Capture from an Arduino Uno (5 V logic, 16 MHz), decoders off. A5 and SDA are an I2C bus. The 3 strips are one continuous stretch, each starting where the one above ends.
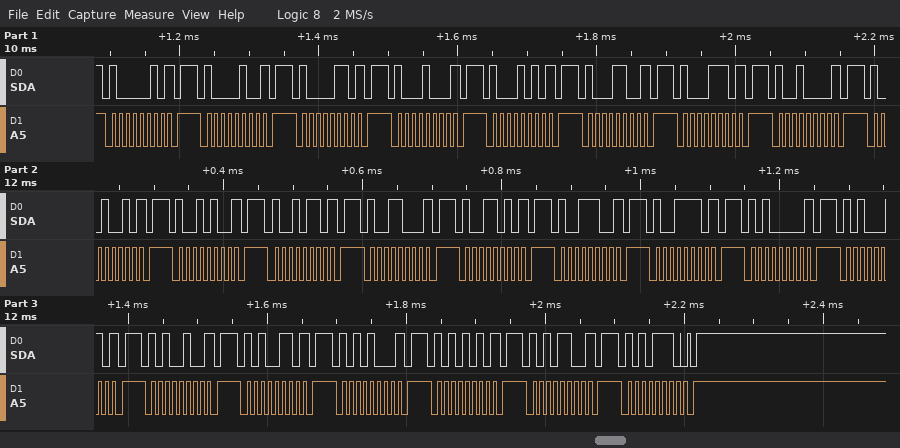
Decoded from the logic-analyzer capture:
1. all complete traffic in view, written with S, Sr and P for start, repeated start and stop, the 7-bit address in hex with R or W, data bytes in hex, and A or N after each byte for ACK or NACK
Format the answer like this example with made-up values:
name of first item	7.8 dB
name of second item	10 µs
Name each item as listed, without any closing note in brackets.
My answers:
all complete traffic in view, written with S, Sr and P for start, repeated start and stop, the 7-bit address in hex with R or W, data bytes in hex, and A or N after each byte for ACK or NACK	S 41W N P S 42W N P S 43W N P S 44W N P S 45W N P S 46W N P S 47W N P S 48W N P S 49W N P S 4AW N P S 4BW N P S 4CW N P S 4DW N P S 4EW N P S 4FW N P S 50W N P S 51W N P S 52W N P S 53W N P S 54W N P S 55W N P S 56W N P S 57W A P
